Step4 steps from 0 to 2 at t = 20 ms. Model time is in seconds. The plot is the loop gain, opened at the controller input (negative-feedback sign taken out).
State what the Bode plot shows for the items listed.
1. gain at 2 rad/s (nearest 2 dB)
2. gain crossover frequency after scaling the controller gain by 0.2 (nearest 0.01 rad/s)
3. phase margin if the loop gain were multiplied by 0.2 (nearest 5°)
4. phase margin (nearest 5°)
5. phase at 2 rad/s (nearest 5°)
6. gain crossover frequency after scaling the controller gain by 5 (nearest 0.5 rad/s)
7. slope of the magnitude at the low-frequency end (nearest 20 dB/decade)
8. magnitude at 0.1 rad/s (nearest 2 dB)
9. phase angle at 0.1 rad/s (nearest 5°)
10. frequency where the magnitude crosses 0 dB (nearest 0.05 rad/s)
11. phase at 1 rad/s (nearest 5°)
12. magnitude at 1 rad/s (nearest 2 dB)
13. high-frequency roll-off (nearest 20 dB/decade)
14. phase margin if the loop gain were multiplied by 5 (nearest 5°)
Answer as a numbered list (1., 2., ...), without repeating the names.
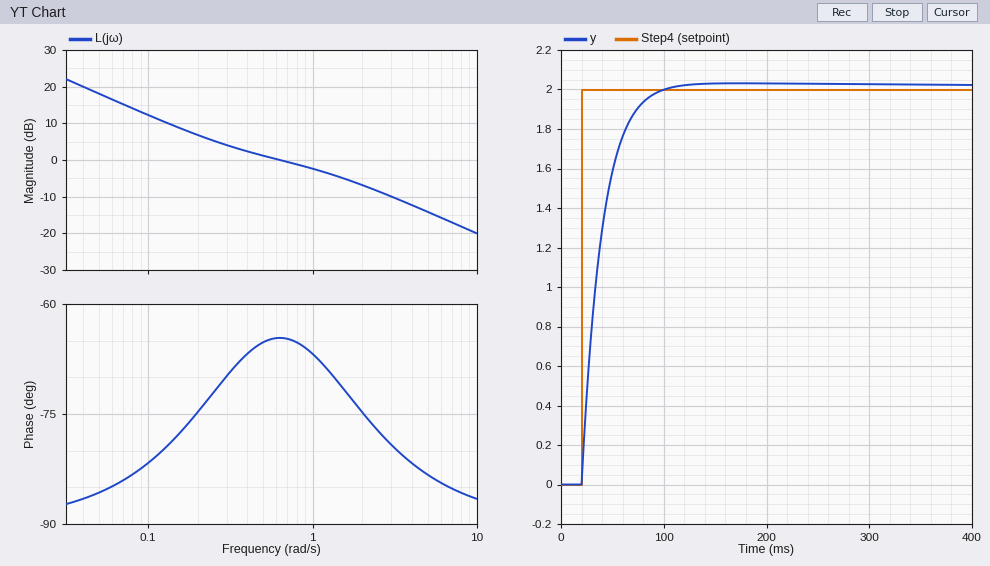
1. -6 dB
2. 0.08 rad/s
3. 95°
4. 115°
5. -75°
6. 5.0 rad/s
7. -20 dB/decade
8. 12 dB
9. -80°
10. 0.65 rad/s
11. -65°
12. -2 dB
13. -20 dB/decade
14. 95°
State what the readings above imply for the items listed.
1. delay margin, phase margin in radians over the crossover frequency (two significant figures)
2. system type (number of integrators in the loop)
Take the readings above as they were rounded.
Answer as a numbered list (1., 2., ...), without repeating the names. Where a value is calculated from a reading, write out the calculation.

1. 115 × π / 180 / 0.65 = 3.1 s
2. 1
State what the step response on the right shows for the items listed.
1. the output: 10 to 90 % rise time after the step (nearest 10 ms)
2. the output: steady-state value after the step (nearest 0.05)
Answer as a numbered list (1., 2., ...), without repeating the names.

1. 40 ms
2. 2.00
